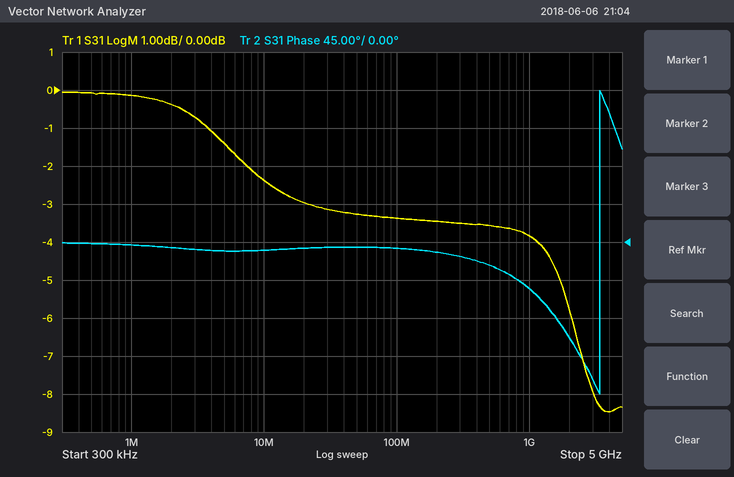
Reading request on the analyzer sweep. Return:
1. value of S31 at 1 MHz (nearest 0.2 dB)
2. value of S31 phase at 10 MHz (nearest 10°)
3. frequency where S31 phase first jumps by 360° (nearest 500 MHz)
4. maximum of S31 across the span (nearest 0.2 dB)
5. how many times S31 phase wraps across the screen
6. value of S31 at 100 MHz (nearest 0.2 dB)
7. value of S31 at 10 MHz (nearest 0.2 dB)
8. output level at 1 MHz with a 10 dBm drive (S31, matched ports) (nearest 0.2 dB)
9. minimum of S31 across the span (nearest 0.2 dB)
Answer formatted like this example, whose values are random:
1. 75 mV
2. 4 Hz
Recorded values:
1. -0.2 dB
2. -10°
3. 3.5 GHz
4. 0.0 dB
5. 1
6. -3.4 dB
7. -2.4 dB
8. 9.8 dBm
9. -8.4 dB
